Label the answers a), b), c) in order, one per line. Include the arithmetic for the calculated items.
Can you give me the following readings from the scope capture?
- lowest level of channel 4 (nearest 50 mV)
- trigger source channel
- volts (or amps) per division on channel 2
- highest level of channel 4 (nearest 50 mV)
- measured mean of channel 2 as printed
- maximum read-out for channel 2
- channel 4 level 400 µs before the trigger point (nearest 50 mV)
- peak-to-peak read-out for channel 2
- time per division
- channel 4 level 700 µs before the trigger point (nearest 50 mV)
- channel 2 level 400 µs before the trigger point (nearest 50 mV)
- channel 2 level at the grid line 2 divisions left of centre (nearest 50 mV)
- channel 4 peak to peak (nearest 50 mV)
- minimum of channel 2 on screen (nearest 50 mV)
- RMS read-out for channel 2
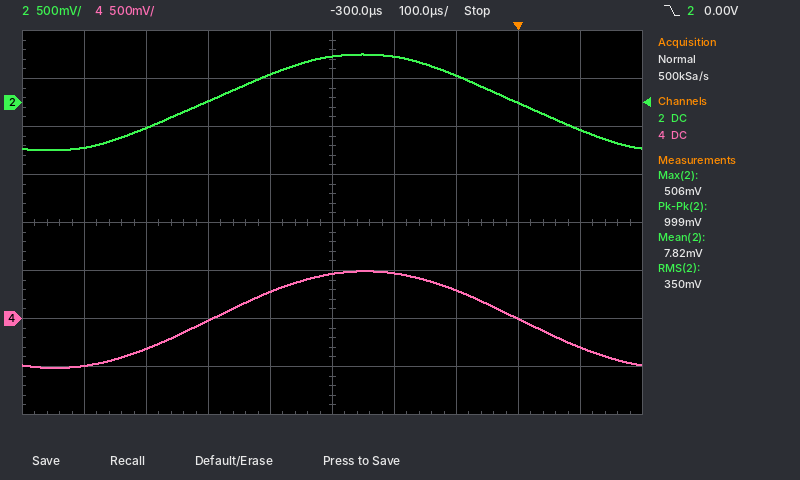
a) -500 mV
b) channel 2
c) 500 mV
d) 500 mV
e) 7.82 mV
f) 506 mV
g) 300 mV
h) 999 mV
i) 100 µs
j) -500 mV
k) 300 mV
l) 0 mV
m) 500 mV − (-500 mV) = 1.00 V
n) -500 mV
o) 350 mV
